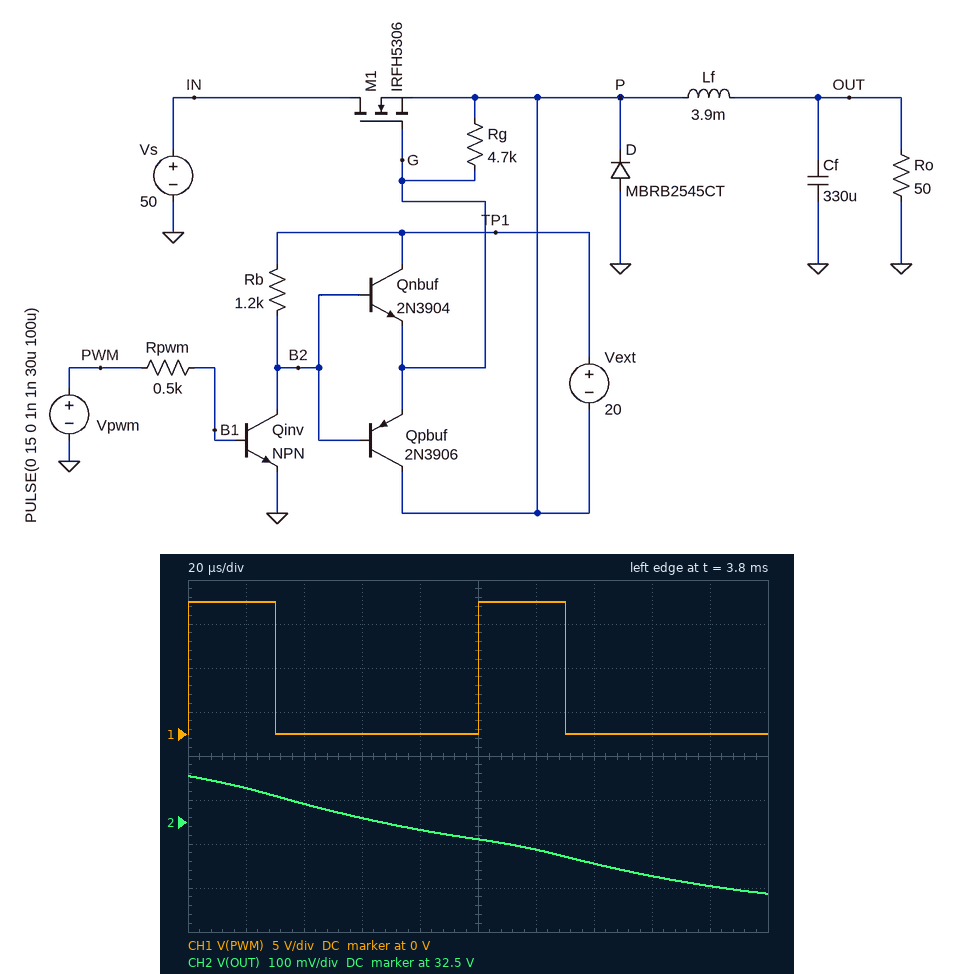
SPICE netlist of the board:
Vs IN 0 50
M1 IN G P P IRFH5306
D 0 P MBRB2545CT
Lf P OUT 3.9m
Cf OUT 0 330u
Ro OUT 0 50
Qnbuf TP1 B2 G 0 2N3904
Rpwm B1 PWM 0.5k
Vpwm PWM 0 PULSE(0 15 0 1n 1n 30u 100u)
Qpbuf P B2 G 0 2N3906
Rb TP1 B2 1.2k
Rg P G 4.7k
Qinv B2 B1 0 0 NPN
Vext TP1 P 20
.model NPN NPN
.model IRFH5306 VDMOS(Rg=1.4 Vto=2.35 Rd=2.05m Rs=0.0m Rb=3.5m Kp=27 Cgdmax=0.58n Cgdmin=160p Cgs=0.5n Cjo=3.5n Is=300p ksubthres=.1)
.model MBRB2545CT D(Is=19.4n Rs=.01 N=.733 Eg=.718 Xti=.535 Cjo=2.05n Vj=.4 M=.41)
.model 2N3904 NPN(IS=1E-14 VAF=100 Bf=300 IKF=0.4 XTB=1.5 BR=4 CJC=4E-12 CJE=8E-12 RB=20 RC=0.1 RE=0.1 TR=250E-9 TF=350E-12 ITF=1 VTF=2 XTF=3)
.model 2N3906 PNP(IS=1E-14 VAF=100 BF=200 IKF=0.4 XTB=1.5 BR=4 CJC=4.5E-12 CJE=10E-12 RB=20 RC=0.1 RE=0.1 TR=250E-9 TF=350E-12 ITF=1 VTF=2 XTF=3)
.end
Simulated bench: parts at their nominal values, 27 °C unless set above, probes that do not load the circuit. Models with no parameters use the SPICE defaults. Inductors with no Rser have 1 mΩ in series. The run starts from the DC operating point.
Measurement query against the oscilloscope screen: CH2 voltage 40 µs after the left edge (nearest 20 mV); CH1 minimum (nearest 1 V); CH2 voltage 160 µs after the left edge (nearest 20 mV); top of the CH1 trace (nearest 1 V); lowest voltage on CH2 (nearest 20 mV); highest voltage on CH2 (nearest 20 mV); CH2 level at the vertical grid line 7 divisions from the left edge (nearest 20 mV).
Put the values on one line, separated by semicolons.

32.54 V; 0 V; 32.38 V; 15 V; 32.34 V; 32.60 V; 32.40 V
